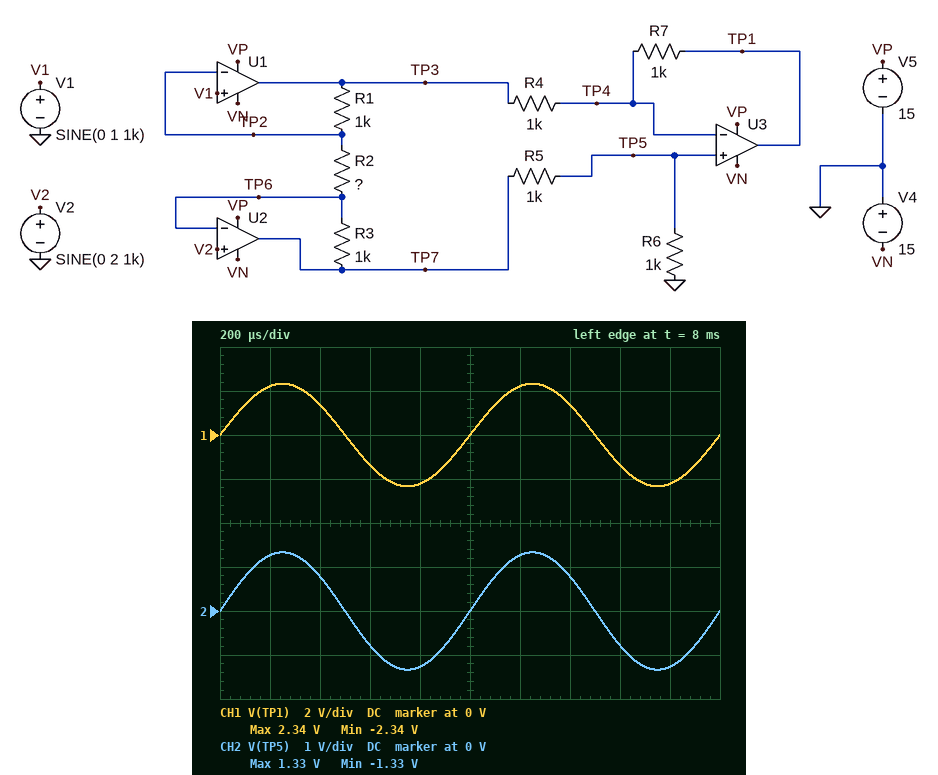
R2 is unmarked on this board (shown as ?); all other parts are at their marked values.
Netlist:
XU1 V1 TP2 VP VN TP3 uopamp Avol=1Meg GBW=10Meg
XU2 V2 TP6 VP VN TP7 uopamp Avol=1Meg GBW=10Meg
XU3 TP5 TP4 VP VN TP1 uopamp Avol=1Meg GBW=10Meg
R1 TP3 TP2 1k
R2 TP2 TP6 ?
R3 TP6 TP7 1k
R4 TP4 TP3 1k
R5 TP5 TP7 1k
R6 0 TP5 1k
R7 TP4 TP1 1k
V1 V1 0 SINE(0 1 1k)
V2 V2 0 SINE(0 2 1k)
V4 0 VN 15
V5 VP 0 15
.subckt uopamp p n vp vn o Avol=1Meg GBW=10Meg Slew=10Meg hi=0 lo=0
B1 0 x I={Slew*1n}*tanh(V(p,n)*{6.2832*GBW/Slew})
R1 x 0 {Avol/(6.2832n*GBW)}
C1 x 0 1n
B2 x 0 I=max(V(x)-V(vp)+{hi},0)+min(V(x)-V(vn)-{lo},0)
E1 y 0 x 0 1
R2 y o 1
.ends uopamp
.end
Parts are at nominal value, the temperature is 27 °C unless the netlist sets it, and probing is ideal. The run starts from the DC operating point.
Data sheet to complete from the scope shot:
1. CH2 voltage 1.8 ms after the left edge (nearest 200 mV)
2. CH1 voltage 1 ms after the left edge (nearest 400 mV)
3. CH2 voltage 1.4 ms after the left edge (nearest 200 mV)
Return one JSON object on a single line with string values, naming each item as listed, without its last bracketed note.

{"CH2 voltage 1.8 ms after the left edge": "-1.2 V", "CH1 voltage 1 ms after the left edge": "0 V", "CH2 voltage 1.4 ms after the left edge": "800 mV"}
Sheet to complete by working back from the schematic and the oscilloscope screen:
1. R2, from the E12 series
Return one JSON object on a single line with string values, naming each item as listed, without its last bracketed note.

{"R2, from the E12 series": "1.5 kΩ"}
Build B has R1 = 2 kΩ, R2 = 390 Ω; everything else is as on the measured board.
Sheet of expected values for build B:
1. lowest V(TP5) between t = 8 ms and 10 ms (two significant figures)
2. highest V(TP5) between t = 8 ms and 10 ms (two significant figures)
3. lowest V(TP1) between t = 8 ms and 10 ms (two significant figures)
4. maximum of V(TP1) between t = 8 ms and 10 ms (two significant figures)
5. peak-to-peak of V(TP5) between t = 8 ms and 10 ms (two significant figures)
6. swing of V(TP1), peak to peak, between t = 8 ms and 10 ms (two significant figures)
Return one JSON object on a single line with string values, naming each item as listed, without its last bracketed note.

{"lowest V(TP5) between t = 8 ms and 10 ms": "-2.3 V", "highest V(TP5) between t = 8 ms and 10 ms": "2.3 V", "lowest V(TP1) between t = 8 ms and 10 ms": "-8.7 V", "maximum of V(TP1) between t = 8 ms and 10 ms": "8.7 V", "peak-to-peak of V(TP5) between t = 8 ms and 10 ms": "4.6 V", "swing of V(TP1), peak to peak, between t = 8 ms and 10 ms": "17 V"}
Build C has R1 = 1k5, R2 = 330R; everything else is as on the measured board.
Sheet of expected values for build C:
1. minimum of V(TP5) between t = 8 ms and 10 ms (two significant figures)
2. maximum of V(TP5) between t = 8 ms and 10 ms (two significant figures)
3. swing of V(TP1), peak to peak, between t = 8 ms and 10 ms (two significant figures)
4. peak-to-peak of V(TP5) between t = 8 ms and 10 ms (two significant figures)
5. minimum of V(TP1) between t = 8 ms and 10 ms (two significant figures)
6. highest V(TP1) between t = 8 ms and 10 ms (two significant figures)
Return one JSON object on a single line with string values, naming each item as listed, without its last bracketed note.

{"minimum of V(TP5) between t = 8 ms and 10 ms": "-2.5 V", "maximum of V(TP5) between t = 8 ms and 10 ms": "2.5 V", "swing of V(TP1), peak to peak, between t = 8 ms and 10 ms": "17 V", "peak-to-peak of V(TP5) between t = 8 ms and 10 ms": "5.0 V", "minimum of V(TP1) between t = 8 ms and 10 ms": "-8.6 V", "highest V(TP1) between t = 8 ms and 10 ms": "8.6 V"}
